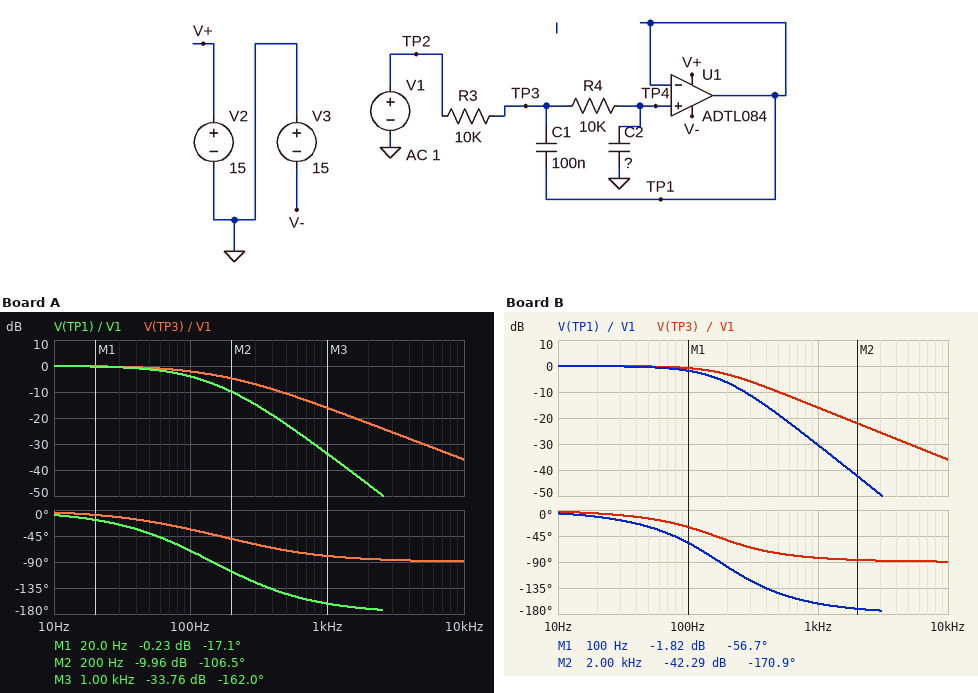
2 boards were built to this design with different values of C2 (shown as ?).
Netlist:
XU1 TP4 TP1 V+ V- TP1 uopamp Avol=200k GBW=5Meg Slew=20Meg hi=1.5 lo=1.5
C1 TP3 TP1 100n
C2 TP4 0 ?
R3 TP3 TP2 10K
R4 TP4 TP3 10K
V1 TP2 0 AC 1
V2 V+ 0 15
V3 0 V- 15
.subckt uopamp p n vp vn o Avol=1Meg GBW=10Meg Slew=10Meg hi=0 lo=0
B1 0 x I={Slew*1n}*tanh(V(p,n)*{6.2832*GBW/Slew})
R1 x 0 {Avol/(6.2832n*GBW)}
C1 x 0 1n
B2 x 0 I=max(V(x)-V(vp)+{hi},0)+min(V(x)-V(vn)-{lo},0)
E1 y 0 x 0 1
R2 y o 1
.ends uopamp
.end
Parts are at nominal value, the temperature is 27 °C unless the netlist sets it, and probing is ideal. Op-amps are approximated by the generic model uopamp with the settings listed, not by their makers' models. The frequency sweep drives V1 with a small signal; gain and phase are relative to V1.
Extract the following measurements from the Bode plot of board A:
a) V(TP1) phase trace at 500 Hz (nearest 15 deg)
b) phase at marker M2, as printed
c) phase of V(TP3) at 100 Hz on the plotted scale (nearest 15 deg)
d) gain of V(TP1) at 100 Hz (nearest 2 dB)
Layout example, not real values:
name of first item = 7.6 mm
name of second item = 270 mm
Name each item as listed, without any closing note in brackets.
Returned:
V(TP1) phase trace at 500 Hz = -150 deg
phase at marker M2, as printed = -106.5 deg
phase of V(TP3) at 100 Hz on the plotted scale = -30 deg
gain of V(TP1) at 100 Hz = -4 dB
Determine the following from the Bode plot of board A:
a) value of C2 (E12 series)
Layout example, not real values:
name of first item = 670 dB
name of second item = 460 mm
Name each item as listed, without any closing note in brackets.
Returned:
value of C2 = 120 nF
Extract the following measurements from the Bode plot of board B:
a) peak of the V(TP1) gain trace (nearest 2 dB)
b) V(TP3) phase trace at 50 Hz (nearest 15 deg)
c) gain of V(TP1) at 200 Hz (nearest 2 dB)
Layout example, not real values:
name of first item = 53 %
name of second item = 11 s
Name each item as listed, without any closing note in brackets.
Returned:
peak of the V(TP1) gain trace = 0 dB
V(TP3) phase trace at 50 Hz = -15 deg
gain of V(TP1) at 200 Hz = -6 dB
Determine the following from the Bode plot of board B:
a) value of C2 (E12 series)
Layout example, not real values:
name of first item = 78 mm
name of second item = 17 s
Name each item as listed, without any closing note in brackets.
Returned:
value of C2 = 82 nF
